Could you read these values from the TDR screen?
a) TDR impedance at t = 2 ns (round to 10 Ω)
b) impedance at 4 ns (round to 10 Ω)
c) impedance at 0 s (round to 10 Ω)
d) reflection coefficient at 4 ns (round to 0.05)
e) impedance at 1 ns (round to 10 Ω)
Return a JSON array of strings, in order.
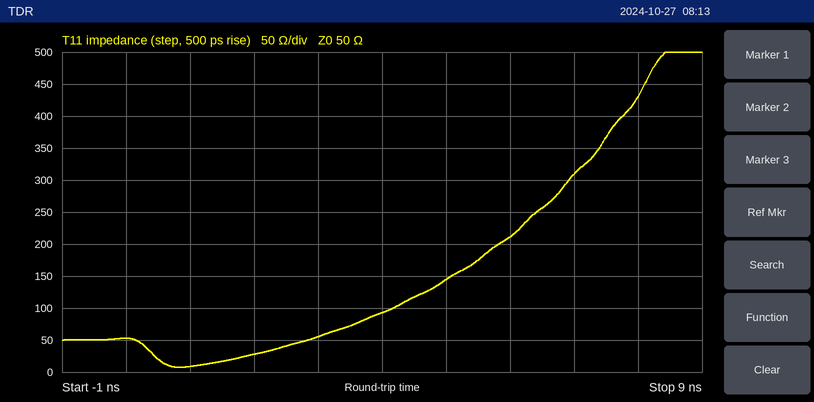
["30 Ω", "90 Ω", "50 Ω", "+0.30", "10 Ω"]
